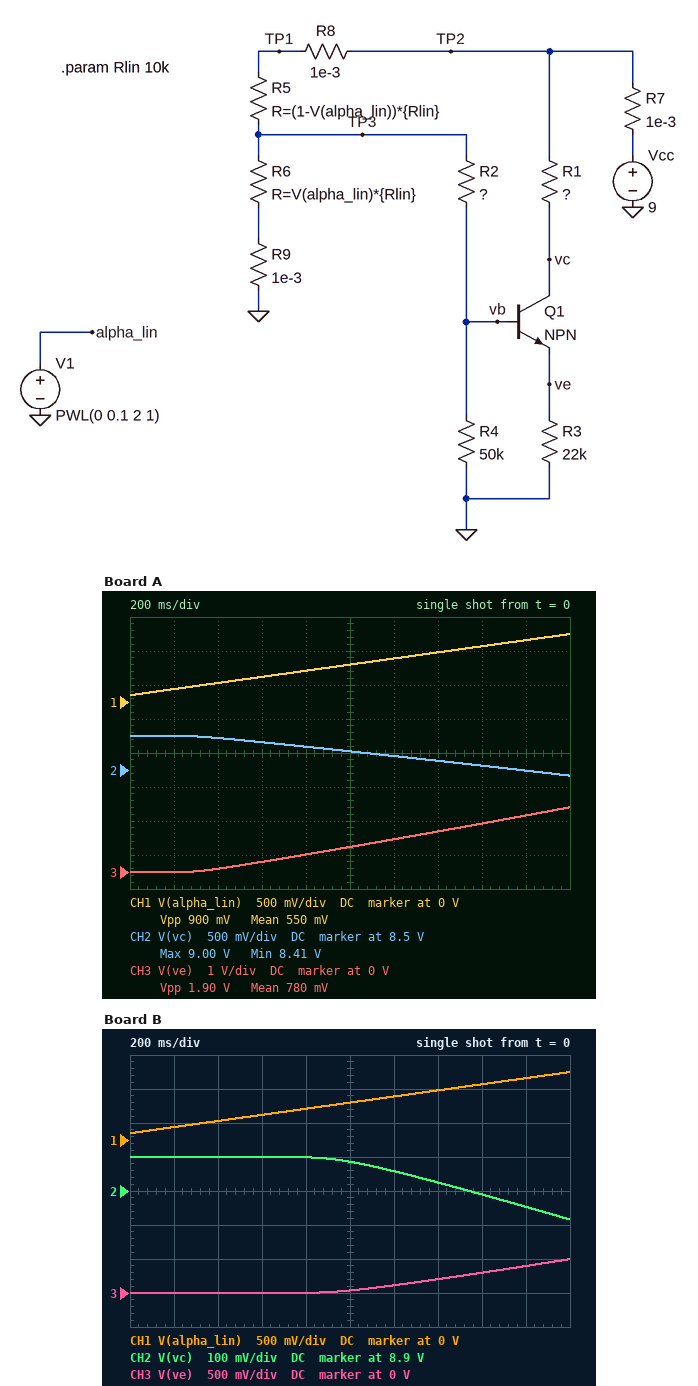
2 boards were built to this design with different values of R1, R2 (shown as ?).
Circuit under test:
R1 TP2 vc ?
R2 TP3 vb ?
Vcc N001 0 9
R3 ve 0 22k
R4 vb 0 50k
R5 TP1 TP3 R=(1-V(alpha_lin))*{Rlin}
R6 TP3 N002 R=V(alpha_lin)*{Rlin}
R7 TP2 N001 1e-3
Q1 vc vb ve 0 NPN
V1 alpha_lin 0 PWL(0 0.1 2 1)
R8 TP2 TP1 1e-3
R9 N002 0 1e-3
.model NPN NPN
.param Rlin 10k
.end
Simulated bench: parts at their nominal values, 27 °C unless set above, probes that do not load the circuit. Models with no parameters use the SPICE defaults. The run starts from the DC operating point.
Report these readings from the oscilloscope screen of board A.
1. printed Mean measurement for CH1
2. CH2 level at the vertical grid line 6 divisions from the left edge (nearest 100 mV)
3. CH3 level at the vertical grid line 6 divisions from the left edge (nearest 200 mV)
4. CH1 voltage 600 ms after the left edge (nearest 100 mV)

550 mV
8.7 V
1.0 V
400 mV
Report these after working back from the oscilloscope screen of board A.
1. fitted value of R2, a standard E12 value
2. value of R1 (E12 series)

120 kΩ
6.8 kΩ
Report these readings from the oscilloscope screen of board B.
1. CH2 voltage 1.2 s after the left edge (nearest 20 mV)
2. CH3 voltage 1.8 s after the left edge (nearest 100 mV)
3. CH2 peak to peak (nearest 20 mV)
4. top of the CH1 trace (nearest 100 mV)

8.96 V
400 mV
180 mV
1.0 V
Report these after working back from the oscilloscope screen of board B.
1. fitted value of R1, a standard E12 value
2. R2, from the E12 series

8.2 kΩ
330 kΩ
